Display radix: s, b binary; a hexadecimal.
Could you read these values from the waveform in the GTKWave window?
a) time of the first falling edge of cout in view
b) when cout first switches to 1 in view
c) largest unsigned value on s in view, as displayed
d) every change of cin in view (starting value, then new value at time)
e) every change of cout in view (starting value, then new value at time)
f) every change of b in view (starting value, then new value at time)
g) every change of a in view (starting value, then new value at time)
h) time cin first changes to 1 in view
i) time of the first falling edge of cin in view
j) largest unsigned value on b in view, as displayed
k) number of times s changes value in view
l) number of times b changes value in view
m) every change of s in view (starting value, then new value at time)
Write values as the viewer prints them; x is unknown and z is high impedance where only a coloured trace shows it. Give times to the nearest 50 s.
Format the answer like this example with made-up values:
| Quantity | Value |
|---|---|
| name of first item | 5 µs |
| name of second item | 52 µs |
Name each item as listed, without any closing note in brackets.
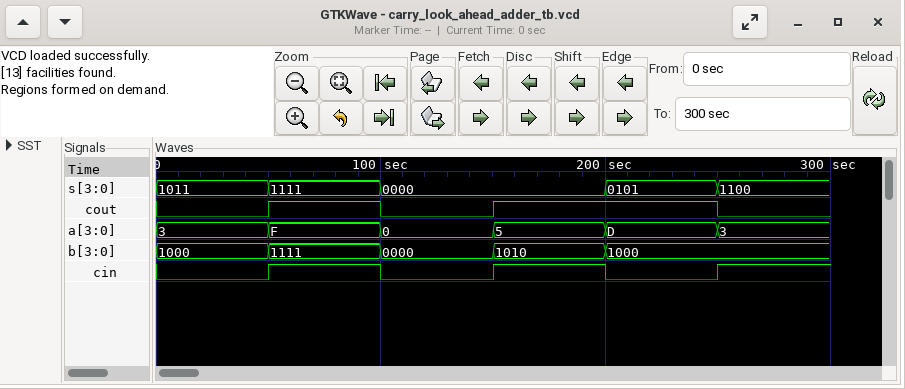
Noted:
| Quantity | Value |
|---|---|
| time of the first falling edge of cout in view | 100 s |
| when cout first switches to 1 in view | 50 s |
| largest unsigned value on s in view, as displayed | 1111 |
| every change of cin in view | 0, 1 at 50 s, 0 at 100 s, 1 at 150 s, 0 at 200 s, 1 at 250 s |
| every change of cout in view | 0, 1 at 50 s, 0 at 100 s, 1 at 150 s, 0 at 250 s |
| every change of b in view | 1000, 1111 at 50 s, 0000 at 100 s, 1010 at 150 s, 1000 at 200 s |
| every change of a in view | 3, F at 50 s, 0 at 100 s, 5 at 150 s, D at 200 s, 3 at 250 s |
| time cin first changes to 1 in view | 50 s |
| time of the first falling edge of cin in view | 100 s |
| largest unsigned value on b in view, as displayed | 1111 |
| number of times s changes value in view | 4 |
| number of times b changes value in view | 4 |
| every change of s in view | 1011, 1111 at 50 s, 0000 at 100 s, 0101 at 200 s, 1100 at 250 s |
